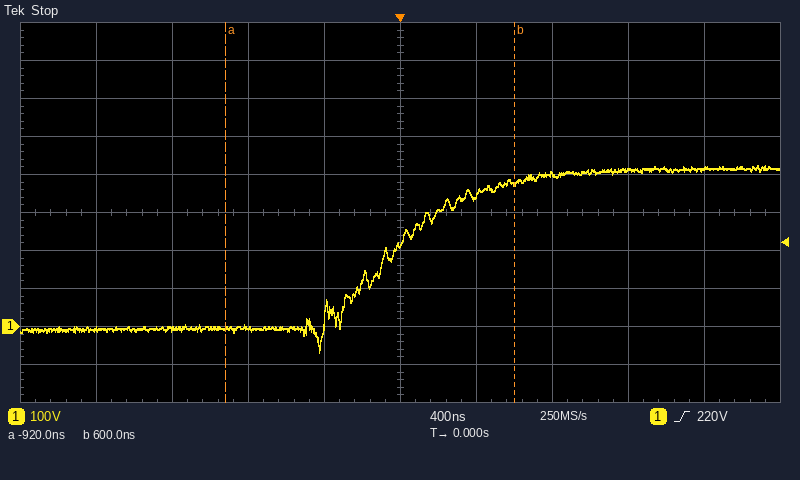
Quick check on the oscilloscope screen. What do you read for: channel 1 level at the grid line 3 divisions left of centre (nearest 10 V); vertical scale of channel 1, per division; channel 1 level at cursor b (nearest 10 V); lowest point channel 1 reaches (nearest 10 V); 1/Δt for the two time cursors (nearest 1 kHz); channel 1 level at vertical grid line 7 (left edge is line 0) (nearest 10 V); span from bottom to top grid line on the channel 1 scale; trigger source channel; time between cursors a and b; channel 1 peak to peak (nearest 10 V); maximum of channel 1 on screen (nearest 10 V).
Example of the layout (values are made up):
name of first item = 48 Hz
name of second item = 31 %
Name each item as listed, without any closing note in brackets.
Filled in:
channel 1 level at the grid line 3 divisions left of centre = -10 V
vertical scale of channel 1, per division = 100 V
channel 1 level at cursor b = 380 V
lowest point channel 1 reaches = -70 V
1/Δt for the two time cursors = 658 kHz
channel 1 level at vertical grid line 7 (left edge is line 0) = 400 V
span from bottom to top grid line on the channel 1 scale = 1 kV
trigger source channel = channel 1
time between cursors a and b = 1.52 µs
channel 1 peak to peak = 490 V
maximum of channel 1 on screen = 420 V
